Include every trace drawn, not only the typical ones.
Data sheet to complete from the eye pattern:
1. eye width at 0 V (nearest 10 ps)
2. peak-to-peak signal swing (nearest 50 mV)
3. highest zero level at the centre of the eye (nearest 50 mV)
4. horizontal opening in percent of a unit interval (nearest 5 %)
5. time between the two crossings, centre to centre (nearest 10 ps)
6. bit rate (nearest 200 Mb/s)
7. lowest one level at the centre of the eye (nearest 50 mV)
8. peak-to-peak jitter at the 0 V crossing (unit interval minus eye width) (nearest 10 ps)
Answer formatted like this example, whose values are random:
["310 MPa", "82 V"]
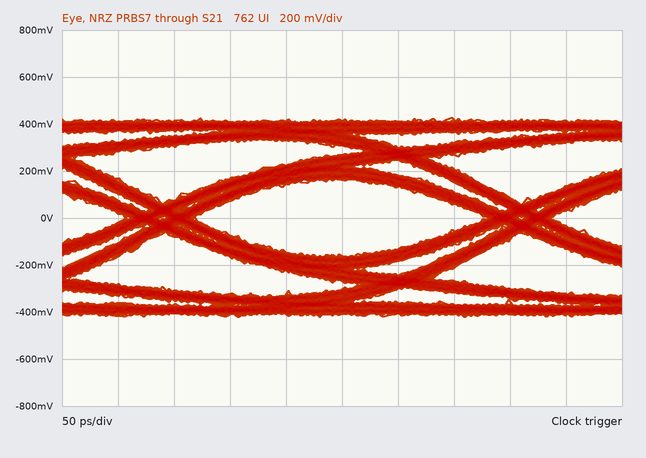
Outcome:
["260 ps", "850 mV", "-150 mV", "80 %", "320 ps", "3.2 Gb/s", "150 mV", "60 ps"]
